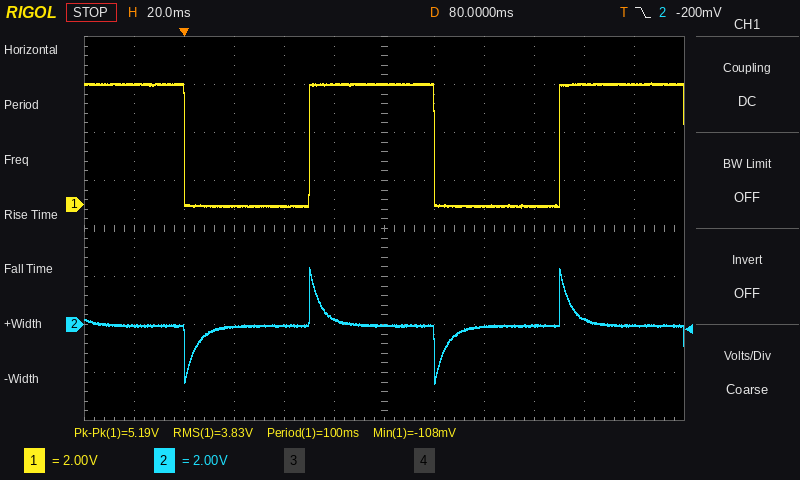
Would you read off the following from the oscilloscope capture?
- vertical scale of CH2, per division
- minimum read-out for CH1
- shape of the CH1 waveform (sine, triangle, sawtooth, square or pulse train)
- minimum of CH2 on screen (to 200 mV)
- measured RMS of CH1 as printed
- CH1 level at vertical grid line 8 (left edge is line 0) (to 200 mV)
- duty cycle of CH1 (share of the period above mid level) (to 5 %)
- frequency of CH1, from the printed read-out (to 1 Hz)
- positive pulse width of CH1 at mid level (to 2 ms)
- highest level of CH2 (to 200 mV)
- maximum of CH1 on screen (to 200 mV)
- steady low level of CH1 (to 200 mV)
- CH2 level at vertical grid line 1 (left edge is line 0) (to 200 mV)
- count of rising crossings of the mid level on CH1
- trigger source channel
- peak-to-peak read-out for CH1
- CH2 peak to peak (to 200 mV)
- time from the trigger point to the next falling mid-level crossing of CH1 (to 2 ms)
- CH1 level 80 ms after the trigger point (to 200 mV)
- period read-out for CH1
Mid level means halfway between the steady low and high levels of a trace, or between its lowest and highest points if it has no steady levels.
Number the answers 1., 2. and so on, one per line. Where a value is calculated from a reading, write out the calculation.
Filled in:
1. 2 V
2. -108 mV
3. square
4. -2.4 V
5. 3.83 V
6. 0.0 V
7. 50 %
8. 1 / 100 ms ≈ 10 Hz
9. 50 ms
10. 2.4 V
11. 5.0 V
12. 0.0 V
13. 0.0 V
14. 2
15. CH2
16. 5.19 V
17. 2.4 V − (-2.4 V) = 4.8 V
18. 100 ms
19. 5.0 V
20. 100 ms
